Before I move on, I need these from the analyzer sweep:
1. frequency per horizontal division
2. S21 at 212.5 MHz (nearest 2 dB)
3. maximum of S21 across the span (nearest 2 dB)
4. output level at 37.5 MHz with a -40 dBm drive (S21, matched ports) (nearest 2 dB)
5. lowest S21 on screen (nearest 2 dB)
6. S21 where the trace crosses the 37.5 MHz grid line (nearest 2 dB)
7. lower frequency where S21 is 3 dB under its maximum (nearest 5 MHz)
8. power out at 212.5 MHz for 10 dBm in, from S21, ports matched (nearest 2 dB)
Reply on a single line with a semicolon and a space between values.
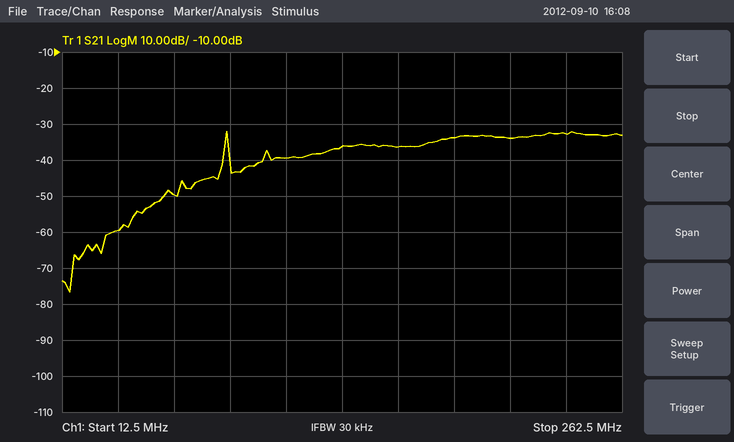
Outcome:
25 MHz; -34 dB; -32 dB; -100 dBm; -76 dB; -60 dB; 85 MHz; -24 dBm
